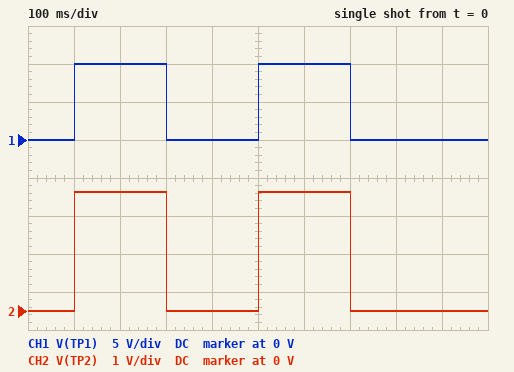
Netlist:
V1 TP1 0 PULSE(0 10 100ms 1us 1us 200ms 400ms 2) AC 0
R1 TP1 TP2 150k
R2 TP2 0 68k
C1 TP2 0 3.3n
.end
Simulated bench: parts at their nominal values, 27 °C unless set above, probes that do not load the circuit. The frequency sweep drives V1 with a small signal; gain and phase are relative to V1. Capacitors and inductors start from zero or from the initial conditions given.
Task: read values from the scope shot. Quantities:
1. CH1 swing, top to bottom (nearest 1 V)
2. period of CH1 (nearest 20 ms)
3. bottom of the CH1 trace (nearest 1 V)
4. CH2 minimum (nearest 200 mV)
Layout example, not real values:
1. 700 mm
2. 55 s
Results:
1. 10 V
2. 400 ms
3. 0 V
4. 0 V
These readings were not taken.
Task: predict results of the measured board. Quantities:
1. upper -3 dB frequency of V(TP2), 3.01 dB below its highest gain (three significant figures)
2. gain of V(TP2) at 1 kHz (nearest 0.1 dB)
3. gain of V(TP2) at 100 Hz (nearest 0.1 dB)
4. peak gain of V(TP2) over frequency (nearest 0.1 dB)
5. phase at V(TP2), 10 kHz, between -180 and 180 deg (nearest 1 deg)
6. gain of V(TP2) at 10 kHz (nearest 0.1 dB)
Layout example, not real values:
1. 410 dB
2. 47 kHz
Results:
1. 1.03 kHz
2. -13.0 dB
3. -10.2 dB
4. -10.1 dB
5. -84 deg
6. -29.9 dB
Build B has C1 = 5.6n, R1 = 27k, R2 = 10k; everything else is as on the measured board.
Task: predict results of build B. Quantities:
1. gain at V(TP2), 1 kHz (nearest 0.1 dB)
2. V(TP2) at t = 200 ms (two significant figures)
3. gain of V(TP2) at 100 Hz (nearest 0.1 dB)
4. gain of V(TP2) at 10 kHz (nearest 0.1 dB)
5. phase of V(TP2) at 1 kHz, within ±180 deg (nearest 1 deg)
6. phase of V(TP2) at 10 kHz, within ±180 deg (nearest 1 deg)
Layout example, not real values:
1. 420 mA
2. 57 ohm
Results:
1. -11.6 dB
2. 2.7 V
3. -11.4 dB
4. -20.2 dB
5. -14 deg
6. -69 deg
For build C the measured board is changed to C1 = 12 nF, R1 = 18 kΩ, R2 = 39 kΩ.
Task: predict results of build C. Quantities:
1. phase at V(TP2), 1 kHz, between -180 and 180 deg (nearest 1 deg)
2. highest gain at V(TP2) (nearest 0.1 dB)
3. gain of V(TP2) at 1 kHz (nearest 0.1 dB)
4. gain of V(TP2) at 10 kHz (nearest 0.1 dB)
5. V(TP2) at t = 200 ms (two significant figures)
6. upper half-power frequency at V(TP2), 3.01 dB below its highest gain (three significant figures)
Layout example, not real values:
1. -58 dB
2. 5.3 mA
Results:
1. -43 deg
2. -3.3 dB
3. -6.0 dB
4. -22.7 dB
5. 6.8 V
6. 1.08 kHz
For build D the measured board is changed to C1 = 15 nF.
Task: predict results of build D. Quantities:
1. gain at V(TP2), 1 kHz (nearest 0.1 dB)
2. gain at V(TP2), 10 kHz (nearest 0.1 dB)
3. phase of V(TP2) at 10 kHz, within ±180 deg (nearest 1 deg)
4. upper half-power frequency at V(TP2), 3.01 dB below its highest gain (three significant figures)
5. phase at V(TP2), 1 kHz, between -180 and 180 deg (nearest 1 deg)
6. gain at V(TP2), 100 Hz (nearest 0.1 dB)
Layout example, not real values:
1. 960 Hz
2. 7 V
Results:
1. -23.2 dB
2. -43.0 dB
3. -89 deg
4. 227 Hz
5. -77 deg
6. -10.9 dB
